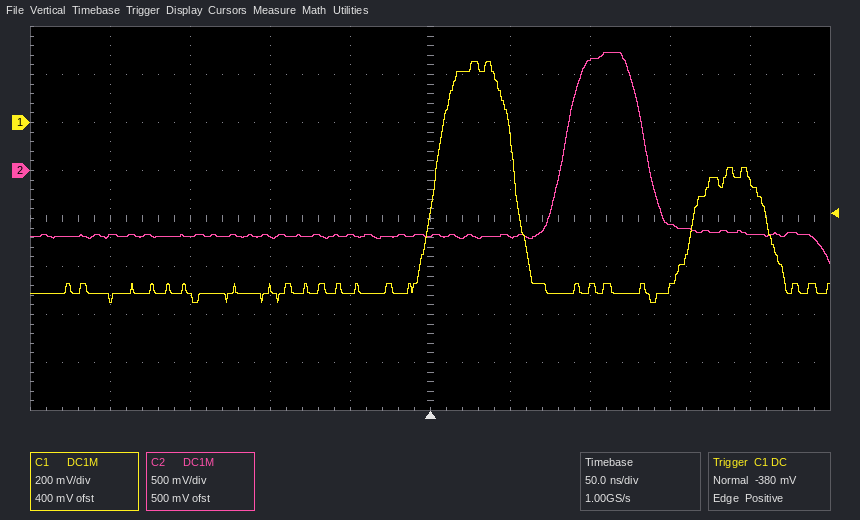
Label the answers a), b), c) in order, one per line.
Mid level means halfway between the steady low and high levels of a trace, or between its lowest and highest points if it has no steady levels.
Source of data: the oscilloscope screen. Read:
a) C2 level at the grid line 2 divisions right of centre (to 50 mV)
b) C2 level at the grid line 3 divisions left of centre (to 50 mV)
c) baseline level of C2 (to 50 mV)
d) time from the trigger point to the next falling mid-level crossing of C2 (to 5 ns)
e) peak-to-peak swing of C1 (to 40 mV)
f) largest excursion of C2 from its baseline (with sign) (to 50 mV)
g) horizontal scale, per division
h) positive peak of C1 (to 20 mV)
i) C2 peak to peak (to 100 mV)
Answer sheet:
a) 1.15 V
b) -700 mV
c) -700 mV
d) 135 ns
e) 1.00 V
f) +1.90 V
g) 50 ns
h) 260 mV
i) 2.20 V
